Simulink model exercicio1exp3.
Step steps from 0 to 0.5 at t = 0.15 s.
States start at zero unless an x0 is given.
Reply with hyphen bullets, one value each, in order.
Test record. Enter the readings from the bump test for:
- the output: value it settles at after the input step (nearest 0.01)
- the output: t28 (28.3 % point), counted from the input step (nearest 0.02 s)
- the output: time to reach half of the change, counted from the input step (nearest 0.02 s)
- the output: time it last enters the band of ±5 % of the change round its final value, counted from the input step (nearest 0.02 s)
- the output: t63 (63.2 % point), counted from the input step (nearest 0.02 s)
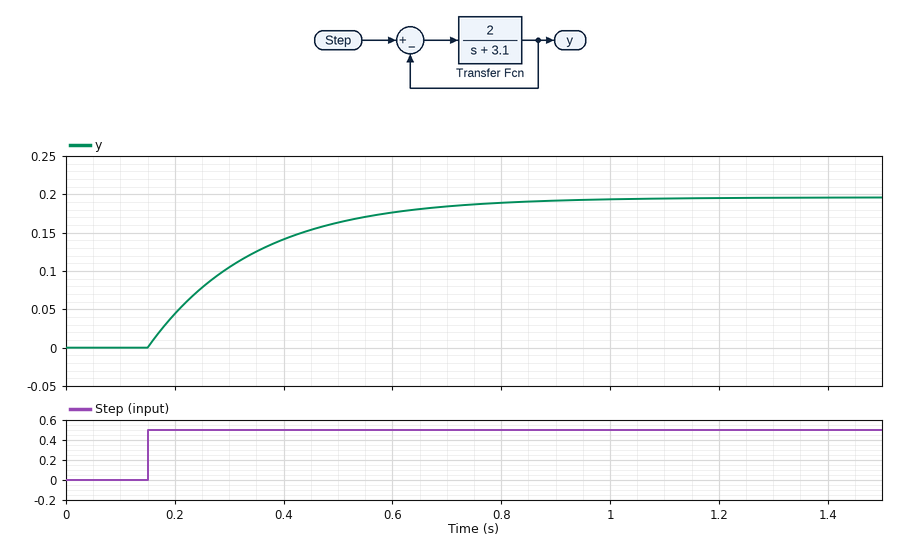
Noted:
- 0.20
- 0.06 s
- 0.14 s
- 0.58 s
- 0.20 s
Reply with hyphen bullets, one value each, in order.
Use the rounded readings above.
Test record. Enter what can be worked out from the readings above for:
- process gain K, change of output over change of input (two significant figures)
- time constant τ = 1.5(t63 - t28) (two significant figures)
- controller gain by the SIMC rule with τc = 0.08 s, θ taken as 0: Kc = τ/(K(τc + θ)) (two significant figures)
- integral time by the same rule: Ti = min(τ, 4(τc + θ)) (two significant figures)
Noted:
- 0.40
- 0.21 s
- 6.6
- 0.21 s
